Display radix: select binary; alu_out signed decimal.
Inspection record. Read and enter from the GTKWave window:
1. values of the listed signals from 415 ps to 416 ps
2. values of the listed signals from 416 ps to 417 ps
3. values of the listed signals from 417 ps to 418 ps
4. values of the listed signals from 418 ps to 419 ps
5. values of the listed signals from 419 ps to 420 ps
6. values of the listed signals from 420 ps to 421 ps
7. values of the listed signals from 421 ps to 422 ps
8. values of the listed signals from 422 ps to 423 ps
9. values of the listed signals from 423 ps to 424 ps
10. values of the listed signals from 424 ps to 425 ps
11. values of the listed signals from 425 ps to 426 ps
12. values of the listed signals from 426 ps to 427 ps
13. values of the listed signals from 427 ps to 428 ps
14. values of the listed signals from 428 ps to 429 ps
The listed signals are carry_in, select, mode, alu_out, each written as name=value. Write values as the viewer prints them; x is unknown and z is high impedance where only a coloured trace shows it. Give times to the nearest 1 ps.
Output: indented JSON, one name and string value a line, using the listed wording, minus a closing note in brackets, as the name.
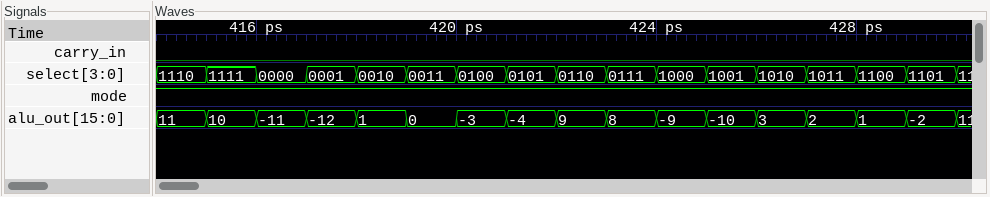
{
  "values of the listed signals from 415 ps to 416 ps": "carry_in=0, select=1111, mode=1, alu_out=10",
  "values of the listed signals from 416 ps to 417 ps": "carry_in=0, select=0000, mode=1, alu_out=-11",
  "values of the listed signals from 417 ps to 418 ps": "carry_in=0, select=0001, mode=1, alu_out=-12",
  "values of the listed signals from 418 ps to 419 ps": "carry_in=0, select=0010, mode=1, alu_out=1",
  "values of the listed signals from 419 ps to 420 ps": "carry_in=0, select=0011, mode=1, alu_out=0",
  "values of the listed signals from 420 ps to 421 ps": "carry_in=0, select=0100, mode=1, alu_out=-3",
  "values of the listed signals from 421 ps to 422 ps": "carry_in=0, select=0101, mode=1, alu_out=-4",
  "values of the listed signals from 422 ps to 423 ps": "carry_in=0, select=0110, mode=1, alu_out=9",
  "values of the listed signals from 423 ps to 424 ps": "carry_in=0, select=0111, mode=1, alu_out=8",
  "values of the listed signals from 424 ps to 425 ps": "carry_in=0, select=1000, mode=1, alu_out=-9",
  "values of the listed signals from 425 ps to 426 ps": "carry_in=0, select=1001, mode=1, alu_out=-10",
  "values of the listed signals from 426 ps to 427 ps": "carry_in=0, select=1010, mode=1, alu_out=3",
  "values of the listed signals from 427 ps to 428 ps": "carry_in=0, select=1011, mode=1, alu_out=2",
  "values of the listed signals from 428 ps to 429 ps": "carry_in=0, select=1100, mode=1, alu_out=1"
}
